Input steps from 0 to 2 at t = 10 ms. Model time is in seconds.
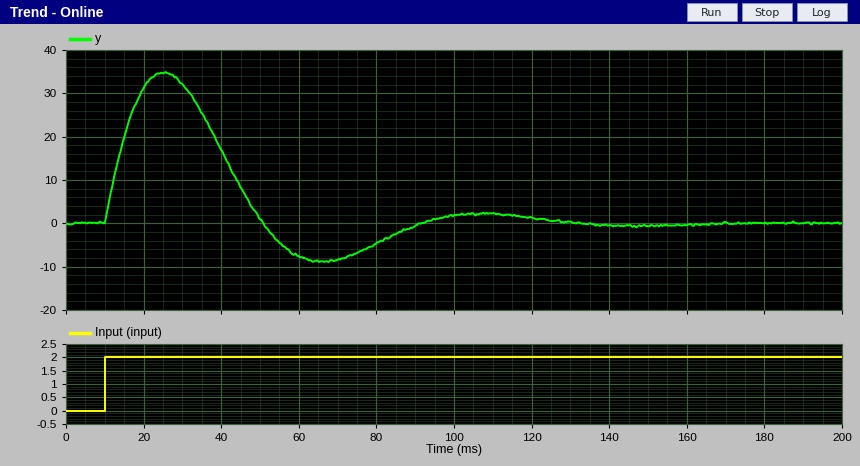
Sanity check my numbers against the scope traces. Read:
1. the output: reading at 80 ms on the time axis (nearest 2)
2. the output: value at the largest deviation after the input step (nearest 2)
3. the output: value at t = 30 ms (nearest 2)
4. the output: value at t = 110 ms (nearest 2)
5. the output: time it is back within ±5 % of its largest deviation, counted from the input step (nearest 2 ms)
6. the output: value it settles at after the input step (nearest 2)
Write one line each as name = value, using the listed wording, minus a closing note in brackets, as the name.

the output: reading at 80 ms on the time axis = -4
the output: value at the largest deviation after the input step = 34
the output: value at t = 30 ms = 32
the output: value at t = 110 ms = 2
the output: time it is back within ±5 % of its largest deviation, counted from the input step = 106 ms
the output: value it settles at after the input step = 0
